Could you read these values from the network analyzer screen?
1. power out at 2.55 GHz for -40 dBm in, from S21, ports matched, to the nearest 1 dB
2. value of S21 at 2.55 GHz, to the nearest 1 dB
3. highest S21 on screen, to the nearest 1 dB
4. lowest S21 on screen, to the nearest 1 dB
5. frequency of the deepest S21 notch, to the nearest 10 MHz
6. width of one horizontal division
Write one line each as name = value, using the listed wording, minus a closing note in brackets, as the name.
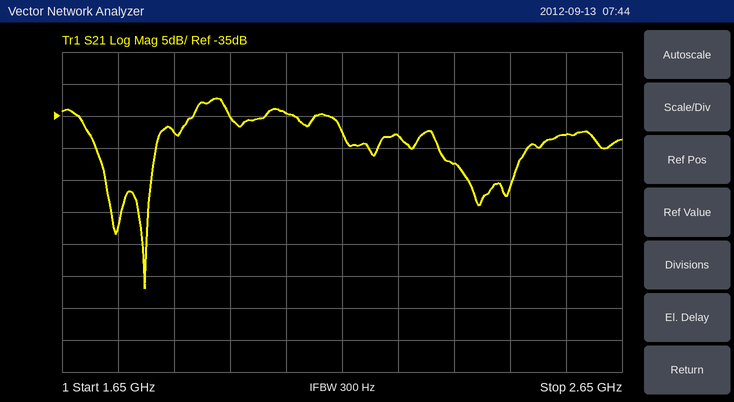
power out at 2.55 GHz for -40 dBm in, from S21, ports matched, to the nearest 1 dB = -78 dBm
value of S21 at 2.55 GHz, to the nearest 1 dB = -38 dB
highest S21 on screen, to the nearest 1 dB = -32 dB
lowest S21 on screen, to the nearest 1 dB = -62 dB
frequency of the deepest S21 notch, to the nearest 10 MHz = 1.80 GHz
width of one horizontal division = 100 MHz
